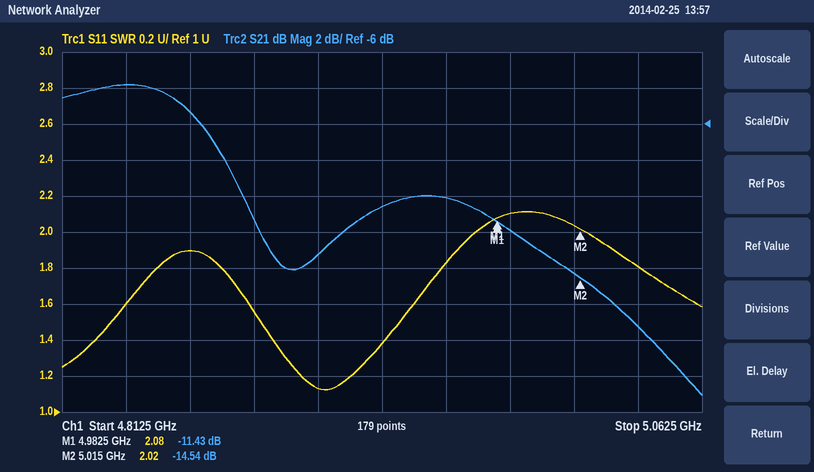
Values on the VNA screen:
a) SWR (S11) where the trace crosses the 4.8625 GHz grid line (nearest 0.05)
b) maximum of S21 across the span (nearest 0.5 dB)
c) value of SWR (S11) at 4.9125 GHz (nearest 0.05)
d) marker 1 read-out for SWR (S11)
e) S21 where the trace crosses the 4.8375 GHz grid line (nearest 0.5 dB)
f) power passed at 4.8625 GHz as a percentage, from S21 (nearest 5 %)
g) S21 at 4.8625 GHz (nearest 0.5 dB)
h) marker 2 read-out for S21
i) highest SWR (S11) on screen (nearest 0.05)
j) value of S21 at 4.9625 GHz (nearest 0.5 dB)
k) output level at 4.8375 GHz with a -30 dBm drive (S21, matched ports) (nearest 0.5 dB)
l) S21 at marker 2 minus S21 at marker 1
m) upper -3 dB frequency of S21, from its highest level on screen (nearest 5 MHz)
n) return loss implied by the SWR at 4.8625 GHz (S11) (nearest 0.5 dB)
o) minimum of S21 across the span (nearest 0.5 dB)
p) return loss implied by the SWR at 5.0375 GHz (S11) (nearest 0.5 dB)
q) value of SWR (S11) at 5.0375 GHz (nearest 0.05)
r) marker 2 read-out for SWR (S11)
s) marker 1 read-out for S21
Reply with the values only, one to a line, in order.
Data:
1.90
-4.0 dB
1.15
2.08
-4.0 dB
30 %
-5.5 dB
-14.54 dB
2.10
-10.0 dB
-34.0 dBm
-3.11 dB
4.870 GHz
10.0 dB
-21.0 dB
11.0 dB
1.80
2.02
-11.43 dB
